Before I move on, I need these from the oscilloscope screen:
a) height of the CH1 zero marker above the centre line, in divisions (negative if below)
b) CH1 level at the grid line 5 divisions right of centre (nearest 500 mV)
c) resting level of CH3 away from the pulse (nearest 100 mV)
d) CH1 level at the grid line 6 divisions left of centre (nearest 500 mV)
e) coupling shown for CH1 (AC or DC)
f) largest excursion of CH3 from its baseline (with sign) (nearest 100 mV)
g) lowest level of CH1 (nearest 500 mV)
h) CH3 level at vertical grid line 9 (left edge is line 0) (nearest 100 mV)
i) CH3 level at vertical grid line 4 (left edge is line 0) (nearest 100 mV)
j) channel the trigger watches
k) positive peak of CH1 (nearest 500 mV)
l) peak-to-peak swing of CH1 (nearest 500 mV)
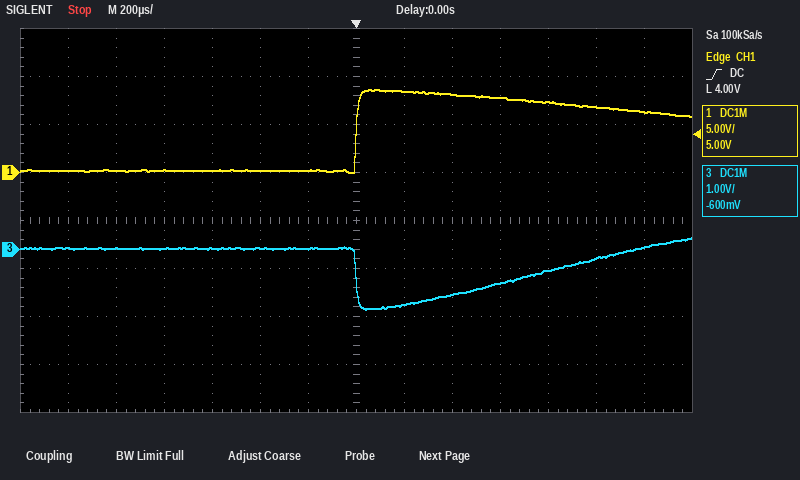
+1.0 div
7.0 V
0.0 V
0.0 V
DC
-1.3 V
0.0 V
-900 mV
0.0 V
CH1
8.5 V
8.5 V
